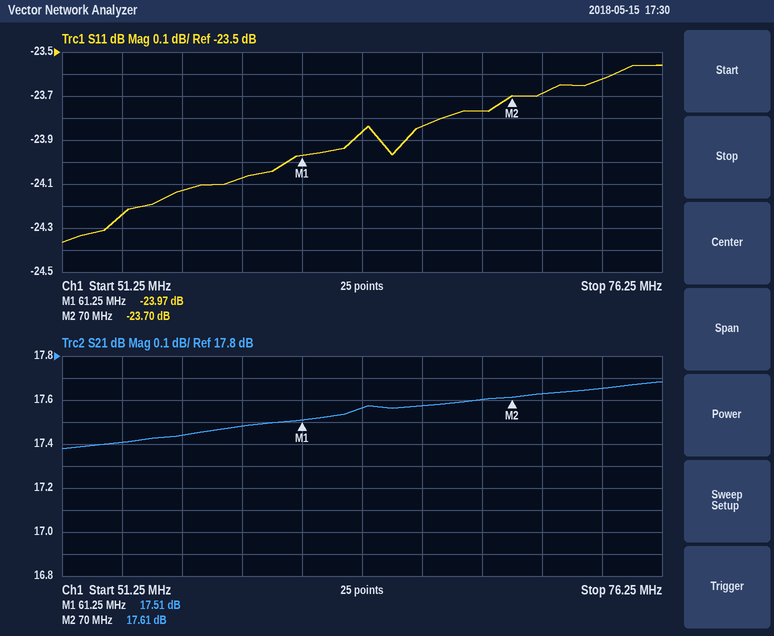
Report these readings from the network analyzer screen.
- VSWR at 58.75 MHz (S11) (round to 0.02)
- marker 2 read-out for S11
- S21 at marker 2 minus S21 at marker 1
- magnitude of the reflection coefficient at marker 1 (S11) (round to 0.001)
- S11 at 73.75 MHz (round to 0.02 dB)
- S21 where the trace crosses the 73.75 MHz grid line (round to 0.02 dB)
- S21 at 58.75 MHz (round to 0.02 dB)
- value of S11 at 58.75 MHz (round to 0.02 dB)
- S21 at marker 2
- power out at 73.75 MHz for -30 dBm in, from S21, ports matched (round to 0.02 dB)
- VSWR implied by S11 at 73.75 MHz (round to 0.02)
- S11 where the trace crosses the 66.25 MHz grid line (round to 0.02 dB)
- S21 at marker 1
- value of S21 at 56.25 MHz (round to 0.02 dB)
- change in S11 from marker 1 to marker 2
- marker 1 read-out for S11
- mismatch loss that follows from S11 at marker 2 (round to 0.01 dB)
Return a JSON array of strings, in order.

["1.14", "-23.70 dB", "0.10 dB", "0.063", "-23.62 dB", "17.66 dB", "17.48 dB", "-24.08 dB", "17.61 dB", "-12.34 dBm", "1.14", "-23.84 dB", "17.51 dB", "17.44 dB", "0.27 dB", "-23.97 dB", "0.02 dB"]
